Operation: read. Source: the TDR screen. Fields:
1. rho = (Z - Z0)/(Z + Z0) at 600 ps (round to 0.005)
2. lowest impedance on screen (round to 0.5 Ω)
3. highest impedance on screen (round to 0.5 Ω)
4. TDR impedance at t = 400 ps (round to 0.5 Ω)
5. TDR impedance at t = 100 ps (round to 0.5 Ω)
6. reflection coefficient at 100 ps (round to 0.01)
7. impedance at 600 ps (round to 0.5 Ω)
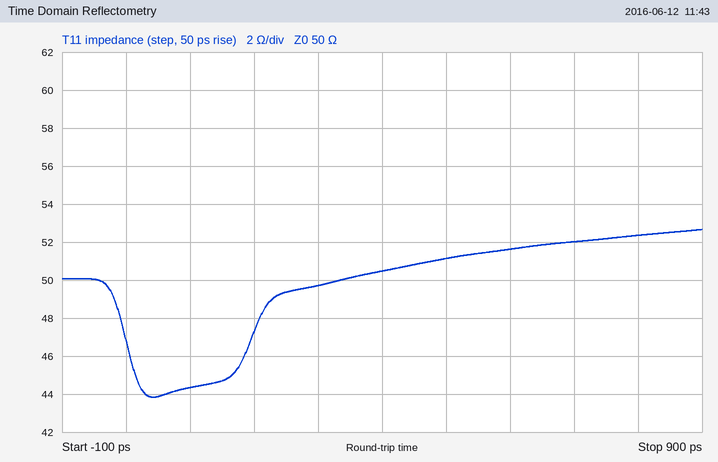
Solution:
+0.015
44.0 Ω
52.5 Ω
50.5 Ω
44.5 Ω
-0.06
51.5 Ω
